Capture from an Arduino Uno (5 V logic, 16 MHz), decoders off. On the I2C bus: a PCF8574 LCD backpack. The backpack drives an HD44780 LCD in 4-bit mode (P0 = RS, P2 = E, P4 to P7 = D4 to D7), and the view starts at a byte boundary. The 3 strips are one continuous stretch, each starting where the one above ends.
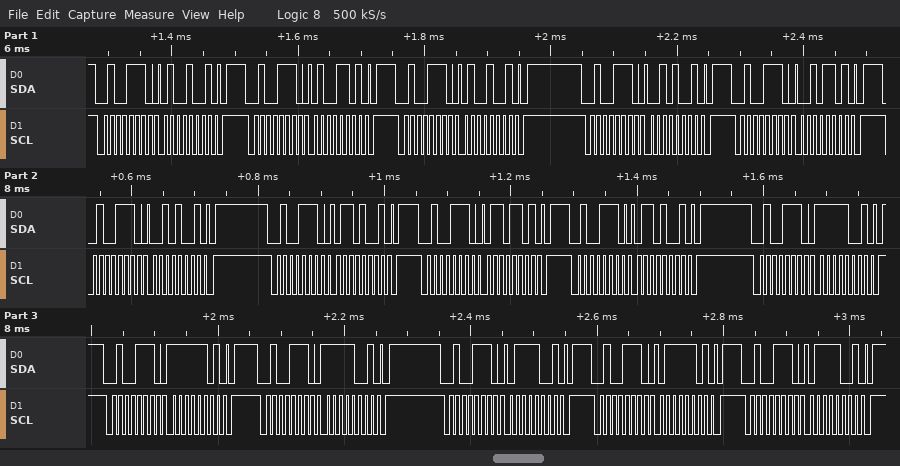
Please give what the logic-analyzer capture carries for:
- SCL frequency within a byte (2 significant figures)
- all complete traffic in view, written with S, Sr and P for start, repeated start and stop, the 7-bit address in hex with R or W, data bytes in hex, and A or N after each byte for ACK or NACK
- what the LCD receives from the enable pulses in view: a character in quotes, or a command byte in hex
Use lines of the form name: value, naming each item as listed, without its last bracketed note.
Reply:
SCL frequency within a byte: 100 kHz
all complete traffic in view, written with S, Sr and P for start, repeated start and stop, the 7-bit address in hex with R or W, data bytes in hex, and A or N after each byte for ACK or NACK: S 27W A 49 A P S 27W A 4D A P S 27W A 49 A P S 27W A 29 A P S 27W A 2D A P S 27W A 29 A P S 27W A 69 A P S 27W A 6D A P S 27W A 69 A P S 27W A F9 A P S 27W A FD A P S 27W A F9 A P S 27W A 79 A P S 27W A 7D A P S 27W A 79 A P
what the LCD receives from the enable pulses in view: a character in quotes, or a command byte in hex: 'B' 'o'
